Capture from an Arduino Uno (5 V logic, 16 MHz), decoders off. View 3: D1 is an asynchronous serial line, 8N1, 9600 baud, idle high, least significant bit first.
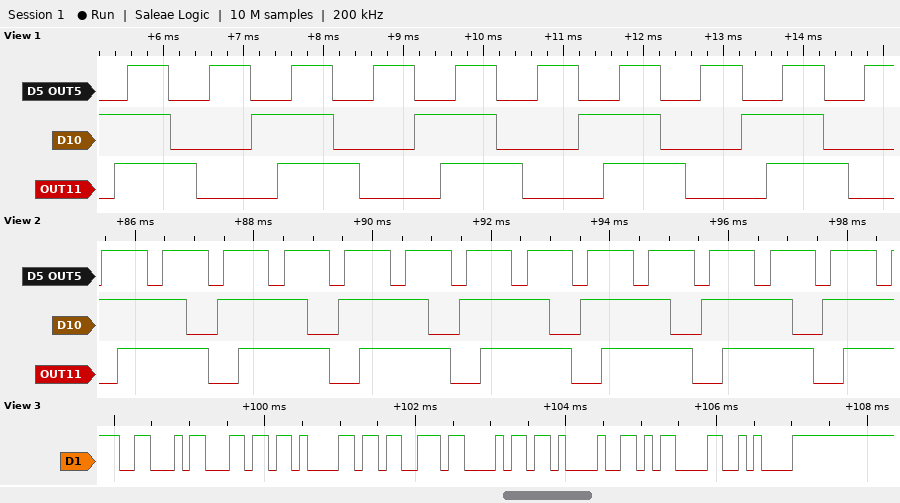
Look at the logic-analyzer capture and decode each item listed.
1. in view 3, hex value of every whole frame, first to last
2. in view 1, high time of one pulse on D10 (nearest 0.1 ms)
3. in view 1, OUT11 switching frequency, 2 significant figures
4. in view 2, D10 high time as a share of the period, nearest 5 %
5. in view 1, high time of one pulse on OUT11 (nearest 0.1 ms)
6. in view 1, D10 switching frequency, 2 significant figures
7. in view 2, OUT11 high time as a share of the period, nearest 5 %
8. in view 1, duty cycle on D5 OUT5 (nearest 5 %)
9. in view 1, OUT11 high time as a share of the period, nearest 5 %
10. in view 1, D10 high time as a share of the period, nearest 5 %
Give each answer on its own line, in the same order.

46 6C 61 73 68 21 0D 0A
1.0 ms
490 Hz
75 %
1.0 ms
490 Hz
75 %
50 %
50 %
50 %
